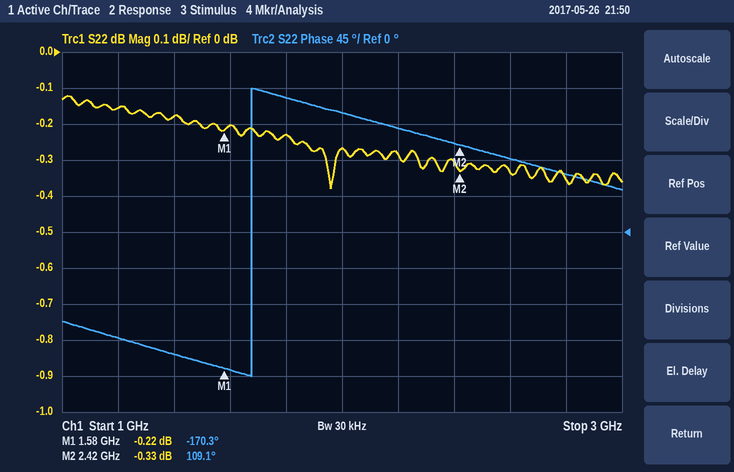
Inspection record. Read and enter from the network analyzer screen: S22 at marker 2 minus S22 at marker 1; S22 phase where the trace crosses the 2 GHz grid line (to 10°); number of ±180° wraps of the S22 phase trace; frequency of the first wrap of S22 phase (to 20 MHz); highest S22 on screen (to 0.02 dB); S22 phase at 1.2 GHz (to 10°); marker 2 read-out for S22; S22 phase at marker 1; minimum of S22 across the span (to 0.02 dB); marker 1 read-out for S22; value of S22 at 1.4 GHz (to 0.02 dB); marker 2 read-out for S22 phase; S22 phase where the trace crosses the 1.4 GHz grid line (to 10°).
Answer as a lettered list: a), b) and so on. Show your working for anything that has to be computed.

a) -0.33 − (-0.22) = -0.11 dB
b) 150°
c) 1
d) 1.68 GHz
e) -0.12 dB
f) -130°
g) -0.33 dB
h) -170.3°
i) -0.38 dB
j) -0.22 dB
k) -0.18 dB
l) 109.1°
m) -150°
